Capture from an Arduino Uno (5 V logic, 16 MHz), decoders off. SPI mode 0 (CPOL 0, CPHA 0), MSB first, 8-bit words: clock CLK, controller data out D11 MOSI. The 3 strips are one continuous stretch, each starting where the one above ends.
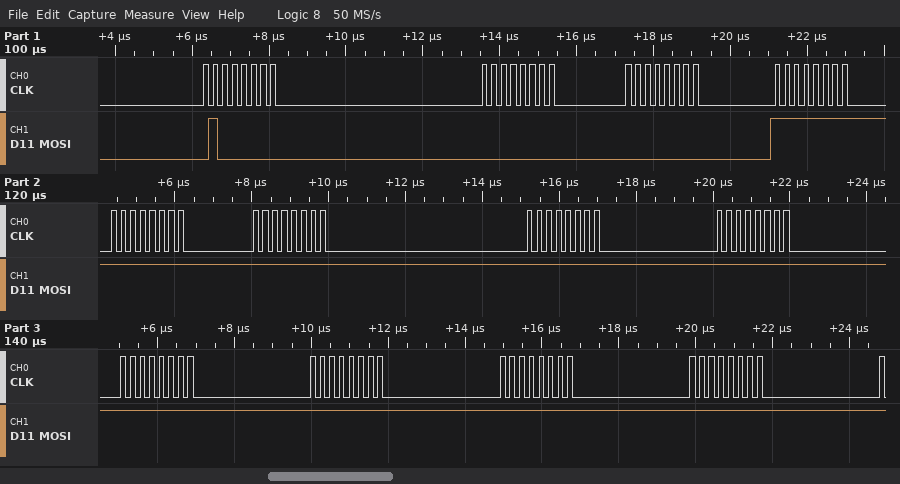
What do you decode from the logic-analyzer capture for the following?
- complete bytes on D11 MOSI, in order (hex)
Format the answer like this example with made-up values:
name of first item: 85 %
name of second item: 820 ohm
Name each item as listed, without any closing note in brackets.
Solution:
complete bytes on D11 MOSI, in order: 40 00 00 FF FF FF FF FF FF FF FF FF
